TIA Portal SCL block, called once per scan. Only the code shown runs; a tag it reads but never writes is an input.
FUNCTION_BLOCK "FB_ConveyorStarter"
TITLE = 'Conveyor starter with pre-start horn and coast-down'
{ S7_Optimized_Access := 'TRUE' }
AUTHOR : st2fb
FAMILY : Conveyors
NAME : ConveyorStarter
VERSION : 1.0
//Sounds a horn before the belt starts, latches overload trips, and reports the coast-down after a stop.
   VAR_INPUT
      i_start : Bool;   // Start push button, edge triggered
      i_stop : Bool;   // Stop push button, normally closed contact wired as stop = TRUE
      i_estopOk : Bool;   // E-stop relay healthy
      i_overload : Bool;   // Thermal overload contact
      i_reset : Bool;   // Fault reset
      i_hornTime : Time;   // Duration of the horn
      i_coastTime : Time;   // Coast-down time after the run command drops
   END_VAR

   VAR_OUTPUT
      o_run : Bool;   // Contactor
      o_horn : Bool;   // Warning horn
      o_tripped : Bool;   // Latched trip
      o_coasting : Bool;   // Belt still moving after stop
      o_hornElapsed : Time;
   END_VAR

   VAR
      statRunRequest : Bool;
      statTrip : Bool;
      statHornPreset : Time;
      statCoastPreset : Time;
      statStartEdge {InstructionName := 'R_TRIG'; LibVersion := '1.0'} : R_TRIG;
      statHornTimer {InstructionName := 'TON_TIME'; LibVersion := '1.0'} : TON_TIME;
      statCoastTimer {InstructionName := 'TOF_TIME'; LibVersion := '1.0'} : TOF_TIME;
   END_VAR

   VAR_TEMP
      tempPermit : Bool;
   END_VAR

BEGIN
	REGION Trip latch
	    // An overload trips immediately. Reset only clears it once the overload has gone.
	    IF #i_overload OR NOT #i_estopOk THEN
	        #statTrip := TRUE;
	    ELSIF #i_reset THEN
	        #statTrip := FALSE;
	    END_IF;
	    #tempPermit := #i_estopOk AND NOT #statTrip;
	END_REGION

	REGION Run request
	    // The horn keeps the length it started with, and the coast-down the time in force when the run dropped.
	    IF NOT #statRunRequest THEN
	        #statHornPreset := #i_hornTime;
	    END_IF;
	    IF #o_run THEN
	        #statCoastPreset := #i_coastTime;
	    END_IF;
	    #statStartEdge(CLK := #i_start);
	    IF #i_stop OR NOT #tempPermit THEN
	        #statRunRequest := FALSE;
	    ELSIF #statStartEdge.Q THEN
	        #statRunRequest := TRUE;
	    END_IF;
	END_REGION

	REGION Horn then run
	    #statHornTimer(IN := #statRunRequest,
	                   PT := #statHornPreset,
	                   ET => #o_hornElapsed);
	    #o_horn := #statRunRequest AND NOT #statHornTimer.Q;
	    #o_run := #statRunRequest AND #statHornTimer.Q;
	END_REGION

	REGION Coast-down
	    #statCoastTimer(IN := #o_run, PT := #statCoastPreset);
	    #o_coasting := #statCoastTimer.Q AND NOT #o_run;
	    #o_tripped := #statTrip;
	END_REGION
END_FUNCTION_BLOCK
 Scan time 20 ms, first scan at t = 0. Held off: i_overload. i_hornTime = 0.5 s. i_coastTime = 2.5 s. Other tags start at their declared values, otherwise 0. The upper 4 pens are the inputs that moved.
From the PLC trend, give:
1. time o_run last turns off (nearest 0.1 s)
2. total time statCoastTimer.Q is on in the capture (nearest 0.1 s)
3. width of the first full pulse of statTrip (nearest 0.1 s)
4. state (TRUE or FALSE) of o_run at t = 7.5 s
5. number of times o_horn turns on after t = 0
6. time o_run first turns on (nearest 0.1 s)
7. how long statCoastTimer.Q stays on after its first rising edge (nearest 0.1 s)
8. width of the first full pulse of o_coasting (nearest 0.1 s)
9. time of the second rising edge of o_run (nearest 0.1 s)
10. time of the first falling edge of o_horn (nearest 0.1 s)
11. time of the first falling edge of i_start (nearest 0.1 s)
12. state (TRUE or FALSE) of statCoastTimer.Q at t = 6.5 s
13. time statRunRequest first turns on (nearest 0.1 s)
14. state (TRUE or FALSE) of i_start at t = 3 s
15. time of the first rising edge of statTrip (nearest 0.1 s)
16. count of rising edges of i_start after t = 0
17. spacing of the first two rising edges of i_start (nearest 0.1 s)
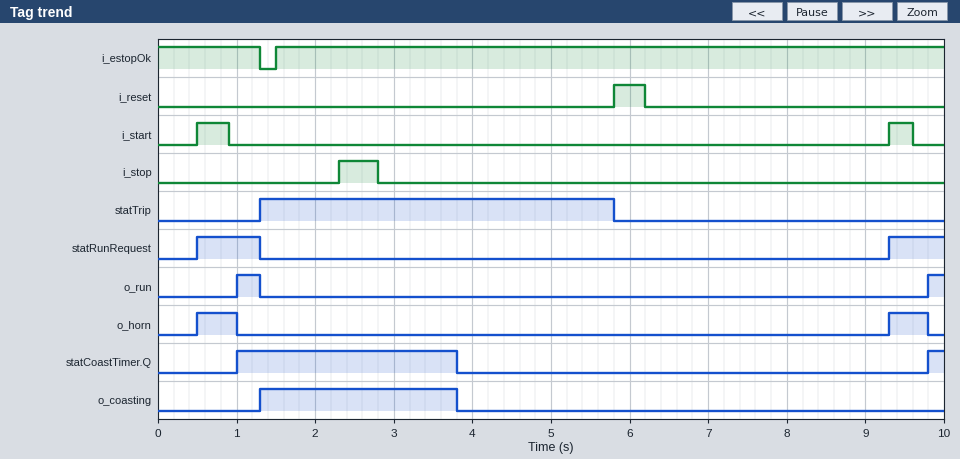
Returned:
1.3 s
3.0 s
4.5 s
FALSE
2
1.0 s
2.8 s
2.5 s
9.8 s
1.0 s
0.9 s
FALSE
0.5 s
FALSE
1.3 s
2
8.8 s
